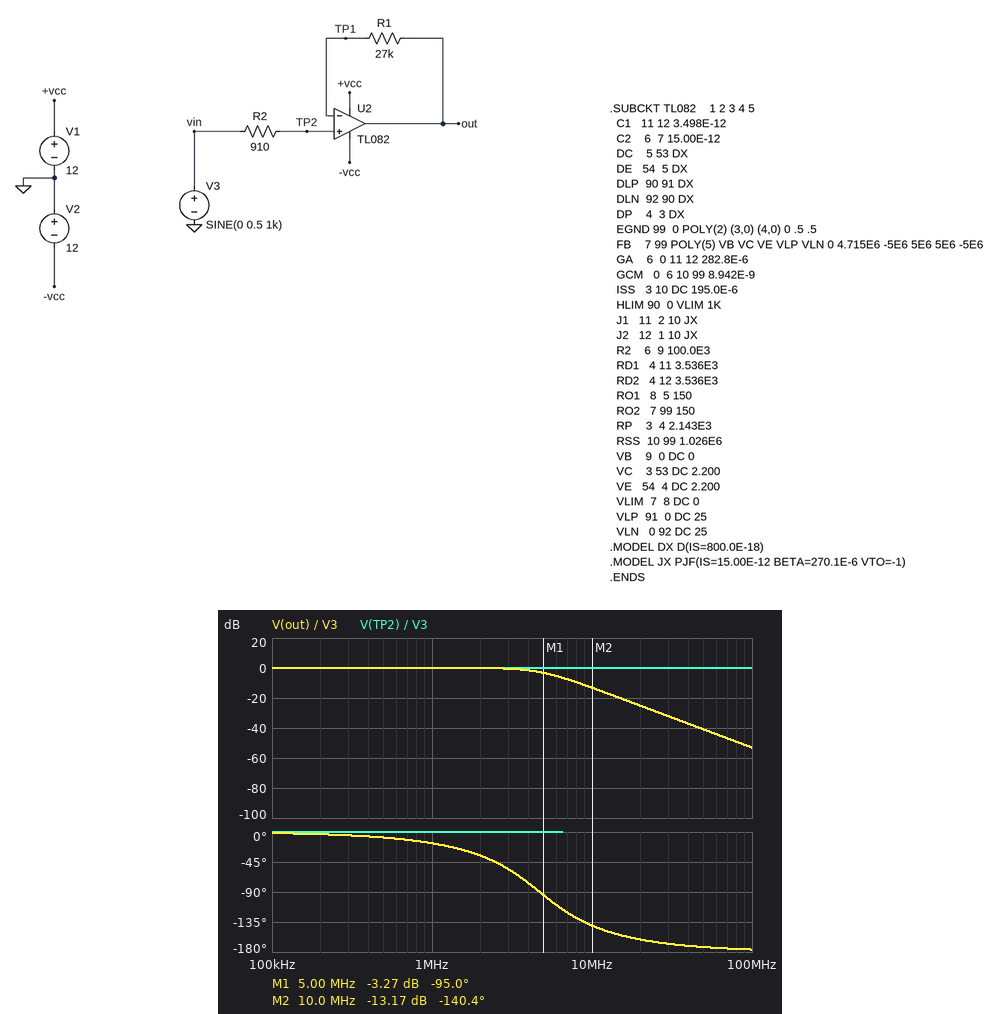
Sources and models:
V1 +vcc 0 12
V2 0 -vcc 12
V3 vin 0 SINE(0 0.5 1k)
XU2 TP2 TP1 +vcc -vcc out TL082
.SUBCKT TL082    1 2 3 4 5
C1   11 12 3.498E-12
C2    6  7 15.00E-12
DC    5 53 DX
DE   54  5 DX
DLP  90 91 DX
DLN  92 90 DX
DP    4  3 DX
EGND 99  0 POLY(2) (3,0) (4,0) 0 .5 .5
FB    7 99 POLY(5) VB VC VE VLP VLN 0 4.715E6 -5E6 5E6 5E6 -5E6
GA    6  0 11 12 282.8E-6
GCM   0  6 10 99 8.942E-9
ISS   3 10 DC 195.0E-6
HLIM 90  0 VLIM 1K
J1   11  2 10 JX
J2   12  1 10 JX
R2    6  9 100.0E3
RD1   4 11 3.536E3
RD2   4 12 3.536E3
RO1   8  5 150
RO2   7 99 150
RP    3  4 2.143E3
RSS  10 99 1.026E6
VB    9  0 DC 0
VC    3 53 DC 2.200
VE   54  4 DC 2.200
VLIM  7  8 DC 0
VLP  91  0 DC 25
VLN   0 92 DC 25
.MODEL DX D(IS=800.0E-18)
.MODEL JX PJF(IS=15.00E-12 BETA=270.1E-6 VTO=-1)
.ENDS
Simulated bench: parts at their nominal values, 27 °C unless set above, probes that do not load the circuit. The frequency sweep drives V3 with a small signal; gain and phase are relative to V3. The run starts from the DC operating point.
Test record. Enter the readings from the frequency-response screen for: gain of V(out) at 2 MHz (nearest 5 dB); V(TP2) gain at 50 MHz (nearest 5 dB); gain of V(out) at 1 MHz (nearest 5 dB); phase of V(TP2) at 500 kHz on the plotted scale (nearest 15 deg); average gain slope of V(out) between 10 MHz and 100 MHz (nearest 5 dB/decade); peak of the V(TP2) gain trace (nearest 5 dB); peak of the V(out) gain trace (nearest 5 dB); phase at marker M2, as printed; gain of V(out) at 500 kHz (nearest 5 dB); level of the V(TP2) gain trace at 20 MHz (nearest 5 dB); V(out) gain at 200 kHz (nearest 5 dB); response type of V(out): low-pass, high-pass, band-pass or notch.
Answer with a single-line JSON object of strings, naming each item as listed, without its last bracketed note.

{"gain of V(out) at 2 MHz": "0 dB", "V(TP2) gain at 50 MHz": "0 dB", "gain of V(out) at 1 MHz": "0 dB", "phase of V(TP2) at 500 kHz on the plotted scale": "0 deg", "average gain slope of V(out) between 10 MHz and 100 MHz": "-40 dB/decade", "peak of the V(TP2) gain trace": "0 dB", "peak of the V(out) gain trace": "0 dB", "phase at marker M2, as printed": "-140.4 deg", "gain of V(out) at 500 kHz": "0 dB", "level of the V(TP2) gain trace at 20 MHz": "0 dB", "V(out) gain at 200 kHz": "0 dB", "response type of V(out): low-pass, high-pass, band-pass or notch": "low-pass"}
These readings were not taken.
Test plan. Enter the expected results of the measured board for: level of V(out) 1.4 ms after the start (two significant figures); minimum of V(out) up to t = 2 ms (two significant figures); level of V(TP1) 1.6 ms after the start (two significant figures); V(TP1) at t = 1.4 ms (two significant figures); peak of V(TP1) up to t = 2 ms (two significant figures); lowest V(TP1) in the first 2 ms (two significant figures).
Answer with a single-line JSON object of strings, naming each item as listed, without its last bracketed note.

{"level of V(out) 1.4 ms after the start": "290 mV", "minimum of V(out) up to t = 2 ms": "-500 mV", "level of V(TP1) 1.6 ms after the start": "-290 mV", "V(TP1) at t = 1.4 ms": "290 mV", "peak of V(TP1) up to t = 2 ms": "500 mV", "lowest V(TP1) in the first 2 ms": "-500 mV"}
